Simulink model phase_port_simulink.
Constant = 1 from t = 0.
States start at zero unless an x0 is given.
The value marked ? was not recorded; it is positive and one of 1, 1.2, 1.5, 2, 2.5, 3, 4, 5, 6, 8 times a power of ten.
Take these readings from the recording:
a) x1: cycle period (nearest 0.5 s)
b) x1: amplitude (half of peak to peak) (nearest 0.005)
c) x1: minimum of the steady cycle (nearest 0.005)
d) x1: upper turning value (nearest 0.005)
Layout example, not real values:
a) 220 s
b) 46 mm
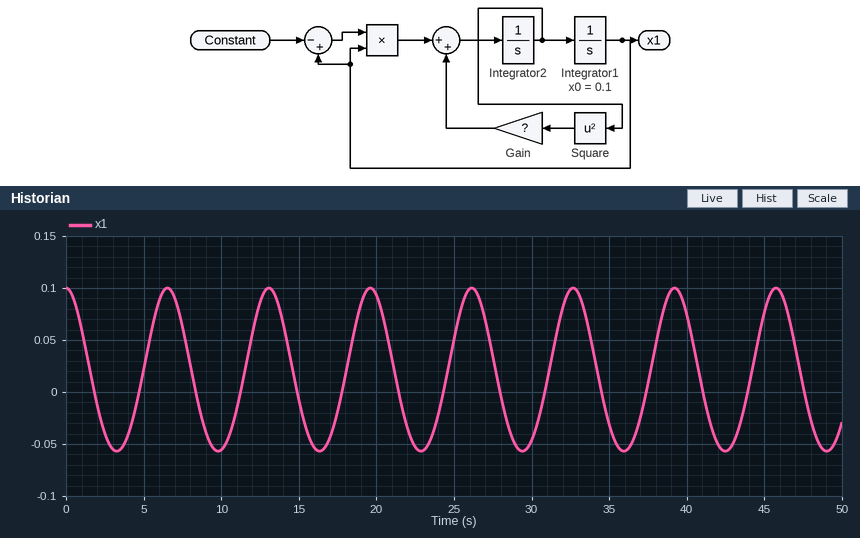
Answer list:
a) 6.5 s
b) 0.080
c) -0.055
d) 0.100
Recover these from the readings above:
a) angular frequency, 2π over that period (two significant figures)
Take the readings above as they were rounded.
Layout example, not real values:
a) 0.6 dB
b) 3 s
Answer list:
a) 0.97 rad/s
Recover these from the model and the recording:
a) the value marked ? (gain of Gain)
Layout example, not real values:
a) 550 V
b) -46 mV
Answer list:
a) 5
